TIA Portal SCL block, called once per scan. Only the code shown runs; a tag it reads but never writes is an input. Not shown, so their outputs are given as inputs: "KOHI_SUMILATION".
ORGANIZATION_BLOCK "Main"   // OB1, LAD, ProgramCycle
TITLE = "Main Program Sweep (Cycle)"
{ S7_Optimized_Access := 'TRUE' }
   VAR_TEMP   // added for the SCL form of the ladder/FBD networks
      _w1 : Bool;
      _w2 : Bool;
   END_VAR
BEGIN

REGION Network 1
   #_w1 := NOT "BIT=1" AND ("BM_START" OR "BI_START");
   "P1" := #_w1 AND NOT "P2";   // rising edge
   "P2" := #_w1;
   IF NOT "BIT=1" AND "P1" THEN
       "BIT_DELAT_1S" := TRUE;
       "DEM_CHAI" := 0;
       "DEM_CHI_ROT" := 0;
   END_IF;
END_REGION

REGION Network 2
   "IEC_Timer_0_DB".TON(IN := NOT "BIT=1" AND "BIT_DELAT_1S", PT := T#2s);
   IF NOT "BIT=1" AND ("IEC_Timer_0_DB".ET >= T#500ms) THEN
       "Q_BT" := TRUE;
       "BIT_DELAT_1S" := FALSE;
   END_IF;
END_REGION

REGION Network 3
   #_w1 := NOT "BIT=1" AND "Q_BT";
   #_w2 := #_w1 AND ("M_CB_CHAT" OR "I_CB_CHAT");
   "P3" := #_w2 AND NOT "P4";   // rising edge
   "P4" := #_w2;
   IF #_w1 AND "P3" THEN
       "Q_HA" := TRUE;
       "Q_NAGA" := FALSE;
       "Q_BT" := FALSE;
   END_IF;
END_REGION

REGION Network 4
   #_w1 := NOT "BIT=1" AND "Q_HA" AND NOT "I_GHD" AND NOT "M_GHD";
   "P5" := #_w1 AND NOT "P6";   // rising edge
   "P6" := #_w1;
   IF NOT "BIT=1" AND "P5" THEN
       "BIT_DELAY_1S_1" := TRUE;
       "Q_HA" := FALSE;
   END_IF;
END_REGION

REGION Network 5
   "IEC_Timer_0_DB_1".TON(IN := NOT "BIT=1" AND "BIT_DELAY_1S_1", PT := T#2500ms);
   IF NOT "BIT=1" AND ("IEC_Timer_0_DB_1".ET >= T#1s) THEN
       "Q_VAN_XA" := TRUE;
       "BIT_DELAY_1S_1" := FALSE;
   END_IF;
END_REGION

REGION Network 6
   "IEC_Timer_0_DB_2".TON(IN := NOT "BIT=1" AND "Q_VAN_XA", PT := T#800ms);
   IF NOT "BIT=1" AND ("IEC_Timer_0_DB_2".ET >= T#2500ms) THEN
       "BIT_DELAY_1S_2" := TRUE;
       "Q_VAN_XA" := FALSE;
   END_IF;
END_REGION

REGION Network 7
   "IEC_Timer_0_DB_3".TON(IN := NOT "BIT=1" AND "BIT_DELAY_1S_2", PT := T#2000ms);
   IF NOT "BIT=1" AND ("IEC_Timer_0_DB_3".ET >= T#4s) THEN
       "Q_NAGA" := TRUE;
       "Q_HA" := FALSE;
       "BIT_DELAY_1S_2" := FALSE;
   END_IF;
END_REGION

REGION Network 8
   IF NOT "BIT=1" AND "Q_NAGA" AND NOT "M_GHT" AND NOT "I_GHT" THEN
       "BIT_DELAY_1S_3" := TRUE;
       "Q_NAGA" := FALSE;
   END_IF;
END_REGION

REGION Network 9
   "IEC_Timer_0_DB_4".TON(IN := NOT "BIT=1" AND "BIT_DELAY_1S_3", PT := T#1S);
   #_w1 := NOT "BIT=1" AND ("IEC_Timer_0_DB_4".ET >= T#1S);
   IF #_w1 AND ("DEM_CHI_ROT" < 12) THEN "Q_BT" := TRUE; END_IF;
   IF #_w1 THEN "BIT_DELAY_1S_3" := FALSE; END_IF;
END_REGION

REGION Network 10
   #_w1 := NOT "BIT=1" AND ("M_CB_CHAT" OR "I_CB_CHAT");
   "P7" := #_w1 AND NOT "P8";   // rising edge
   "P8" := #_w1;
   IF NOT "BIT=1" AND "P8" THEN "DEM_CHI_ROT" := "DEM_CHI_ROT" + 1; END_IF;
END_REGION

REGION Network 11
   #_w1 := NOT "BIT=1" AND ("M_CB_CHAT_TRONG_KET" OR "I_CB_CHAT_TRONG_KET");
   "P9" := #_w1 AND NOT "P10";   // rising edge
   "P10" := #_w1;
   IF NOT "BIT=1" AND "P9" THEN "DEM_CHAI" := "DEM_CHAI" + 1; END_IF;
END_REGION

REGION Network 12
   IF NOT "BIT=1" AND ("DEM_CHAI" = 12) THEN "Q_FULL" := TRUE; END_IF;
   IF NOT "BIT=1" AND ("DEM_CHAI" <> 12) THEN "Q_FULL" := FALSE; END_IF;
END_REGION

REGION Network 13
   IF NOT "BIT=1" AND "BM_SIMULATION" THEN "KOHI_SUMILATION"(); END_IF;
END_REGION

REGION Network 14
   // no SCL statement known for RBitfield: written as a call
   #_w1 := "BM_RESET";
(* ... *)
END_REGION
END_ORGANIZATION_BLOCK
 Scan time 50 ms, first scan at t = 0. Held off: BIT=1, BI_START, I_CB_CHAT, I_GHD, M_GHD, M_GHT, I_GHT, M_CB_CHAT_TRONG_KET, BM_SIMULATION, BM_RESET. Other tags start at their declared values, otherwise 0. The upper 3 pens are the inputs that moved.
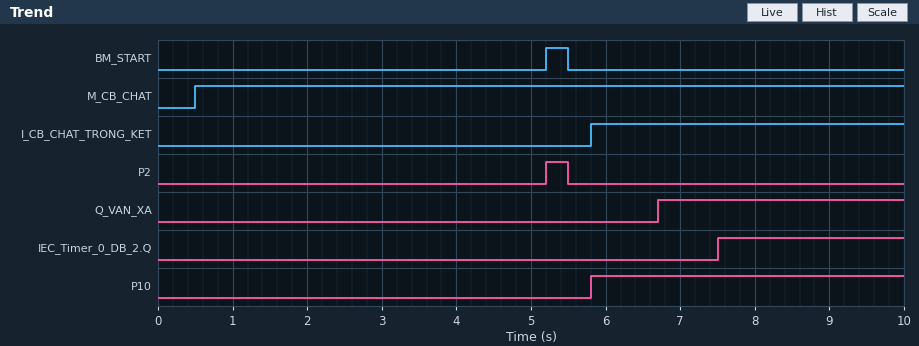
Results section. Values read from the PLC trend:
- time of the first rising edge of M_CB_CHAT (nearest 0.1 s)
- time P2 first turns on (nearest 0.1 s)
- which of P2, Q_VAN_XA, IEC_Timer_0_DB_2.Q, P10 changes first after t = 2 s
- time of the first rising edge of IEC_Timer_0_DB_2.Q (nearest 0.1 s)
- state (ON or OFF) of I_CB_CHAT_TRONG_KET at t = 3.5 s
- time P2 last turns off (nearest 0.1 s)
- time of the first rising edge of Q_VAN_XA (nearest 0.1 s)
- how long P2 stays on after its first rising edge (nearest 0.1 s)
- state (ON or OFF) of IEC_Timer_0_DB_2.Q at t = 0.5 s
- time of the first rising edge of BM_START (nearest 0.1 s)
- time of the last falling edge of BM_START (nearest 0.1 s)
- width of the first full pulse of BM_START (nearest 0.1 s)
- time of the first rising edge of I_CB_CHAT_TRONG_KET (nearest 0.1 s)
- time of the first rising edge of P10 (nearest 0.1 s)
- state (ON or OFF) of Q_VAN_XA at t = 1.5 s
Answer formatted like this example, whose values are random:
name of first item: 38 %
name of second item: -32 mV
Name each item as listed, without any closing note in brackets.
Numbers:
time of the first rising edge of M_CB_CHAT: 0.5 s
time P2 first turns on: 5.2 s
which of P2, Q_VAN_XA, IEC_Timer_0_DB_2.Q, P10 changes first after t = 2 s: P2
time of the first rising edge of IEC_Timer_0_DB_2.Q: 7.5 s
state (ON or OFF) of I_CB_CHAT_TRONG_KET at t = 3.5 s: OFF
time P2 last turns off: 5.5 s
time of the first rising edge of Q_VAN_XA: 6.7 s
how long P2 stays on after its first rising edge: 0.3 s
state (ON or OFF) of IEC_Timer_0_DB_2.Q at t = 0.5 s: OFF
time of the first rising edge of BM_START: 5.2 s
time of the last falling edge of BM_START: 5.5 s
width of the first full pulse of BM_START: 0.3 s
time of the first rising edge of I_CB_CHAT_TRONG_KET: 5.8 s
time of the first rising edge of P10: 5.8 s
state (ON or OFF) of Q_VAN_XA at t = 1.5 s: OFF
